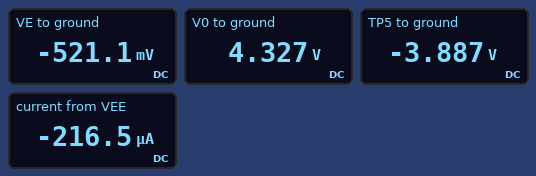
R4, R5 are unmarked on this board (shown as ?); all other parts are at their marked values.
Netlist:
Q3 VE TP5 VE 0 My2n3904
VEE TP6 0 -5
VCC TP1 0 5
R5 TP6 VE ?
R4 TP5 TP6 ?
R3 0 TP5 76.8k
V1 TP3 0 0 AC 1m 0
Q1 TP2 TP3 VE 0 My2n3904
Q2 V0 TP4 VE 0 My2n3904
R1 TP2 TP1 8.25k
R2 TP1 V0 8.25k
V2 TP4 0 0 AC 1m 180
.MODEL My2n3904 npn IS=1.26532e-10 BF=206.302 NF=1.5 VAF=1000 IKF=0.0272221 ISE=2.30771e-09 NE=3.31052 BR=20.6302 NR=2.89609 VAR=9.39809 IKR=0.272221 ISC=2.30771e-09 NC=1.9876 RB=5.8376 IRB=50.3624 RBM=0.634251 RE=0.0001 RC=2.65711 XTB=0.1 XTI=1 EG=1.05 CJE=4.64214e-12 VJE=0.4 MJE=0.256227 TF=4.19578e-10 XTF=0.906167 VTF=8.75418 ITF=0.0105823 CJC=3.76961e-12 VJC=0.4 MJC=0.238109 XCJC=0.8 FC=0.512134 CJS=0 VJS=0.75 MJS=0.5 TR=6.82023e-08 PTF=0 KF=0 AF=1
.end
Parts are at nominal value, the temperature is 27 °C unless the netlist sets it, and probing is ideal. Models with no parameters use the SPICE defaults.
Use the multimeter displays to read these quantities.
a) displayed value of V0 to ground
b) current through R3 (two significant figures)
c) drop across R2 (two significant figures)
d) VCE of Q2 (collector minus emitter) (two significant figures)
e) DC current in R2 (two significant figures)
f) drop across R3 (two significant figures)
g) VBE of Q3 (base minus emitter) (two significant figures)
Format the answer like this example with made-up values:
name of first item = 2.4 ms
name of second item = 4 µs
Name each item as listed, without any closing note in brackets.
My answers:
displayed value of V0 to ground = 4.327 V
current through R3 = 51 µA
drop across R2 = 670 mV
VCE of Q2 (collector minus emitter) = 4.8 V
DC current in R2 = 82 µA
drop across R3 = 3.9 V
VBE of Q3 (base minus emitter) = -3.4 V
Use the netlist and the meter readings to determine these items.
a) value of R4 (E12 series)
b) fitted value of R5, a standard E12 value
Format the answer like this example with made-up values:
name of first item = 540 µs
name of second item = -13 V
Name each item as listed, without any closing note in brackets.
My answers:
value of R4 = 22 kΩ
fitted value of R5, a standard E12 value = 27 kΩ
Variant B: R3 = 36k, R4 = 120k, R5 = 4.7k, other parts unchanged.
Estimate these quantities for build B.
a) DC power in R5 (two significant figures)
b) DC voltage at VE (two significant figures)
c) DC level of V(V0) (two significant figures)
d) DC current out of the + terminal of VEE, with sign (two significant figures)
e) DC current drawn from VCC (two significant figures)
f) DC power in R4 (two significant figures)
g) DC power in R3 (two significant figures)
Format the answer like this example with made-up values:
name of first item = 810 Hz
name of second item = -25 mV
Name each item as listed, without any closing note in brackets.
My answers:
DC power in R5 = 4.1 mW
DC voltage at VE = -590 mV
DC level of V(V0) = 1.2 V
DC current out of the + terminal of VEE, with sign = -970 µA
DC current drawn from VCC = 930 µA
DC power in R4 = 120 µW
DC power in R3 = 37 µW
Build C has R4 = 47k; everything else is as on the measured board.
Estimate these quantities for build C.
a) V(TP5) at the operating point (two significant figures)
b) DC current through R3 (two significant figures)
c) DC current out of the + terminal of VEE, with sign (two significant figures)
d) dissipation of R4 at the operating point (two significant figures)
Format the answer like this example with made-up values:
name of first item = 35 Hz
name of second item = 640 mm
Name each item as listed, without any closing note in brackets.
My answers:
V(TP5) at the operating point = -3.1 V
DC current through R3 = 40 µA
DC current out of the + terminal of VEE, with sign = -210 µA
dissipation of R4 at the operating point = 77 µW
